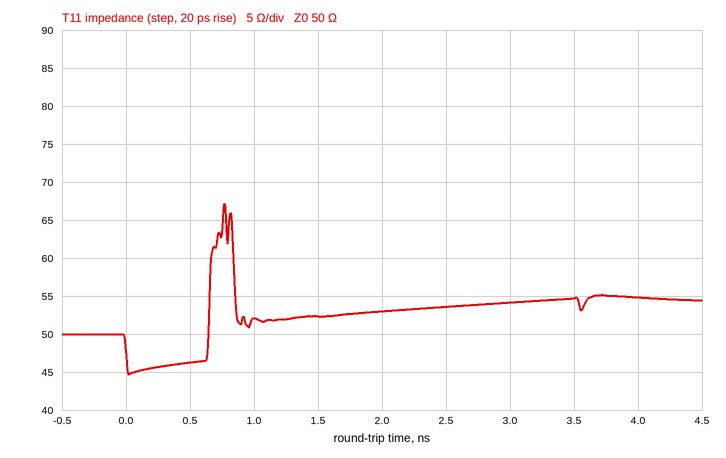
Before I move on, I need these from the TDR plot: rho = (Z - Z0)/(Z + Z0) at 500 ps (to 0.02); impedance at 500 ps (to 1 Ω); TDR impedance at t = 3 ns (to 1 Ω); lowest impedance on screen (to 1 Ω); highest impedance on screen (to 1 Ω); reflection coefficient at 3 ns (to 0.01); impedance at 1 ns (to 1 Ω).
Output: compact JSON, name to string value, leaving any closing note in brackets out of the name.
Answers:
{"rho = (Z - Z0)/(Z + Z0) at 500 ps": "-0.04", "impedance at 500 ps": "46 Ω", "TDR impedance at t = 3 ns": "54 Ω", "lowest impedance on screen": "45 Ω", "highest impedance on screen": "67 Ω", "reflection coefficient at 3 ns": "+0.04", "impedance at 1 ns": "52 Ω"}
